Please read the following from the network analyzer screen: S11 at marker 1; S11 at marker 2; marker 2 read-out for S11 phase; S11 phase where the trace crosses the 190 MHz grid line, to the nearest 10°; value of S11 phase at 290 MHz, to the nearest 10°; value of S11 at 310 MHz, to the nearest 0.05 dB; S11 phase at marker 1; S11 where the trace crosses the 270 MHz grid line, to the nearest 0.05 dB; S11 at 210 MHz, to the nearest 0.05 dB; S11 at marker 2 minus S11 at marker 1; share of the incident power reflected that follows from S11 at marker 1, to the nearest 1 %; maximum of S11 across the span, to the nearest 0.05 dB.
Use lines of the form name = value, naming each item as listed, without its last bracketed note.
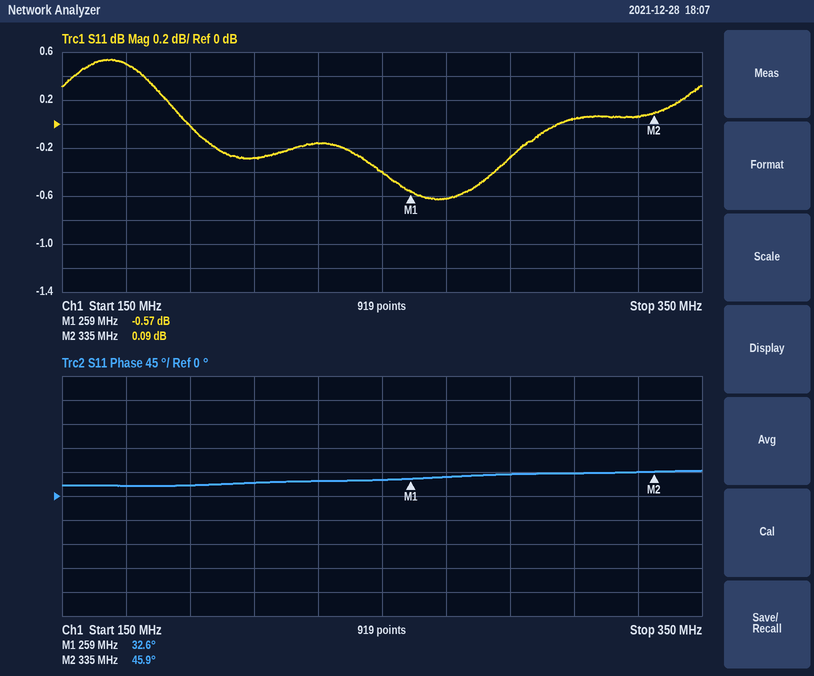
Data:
S11 at marker 1 = -0.57 dB
S11 at marker 2 = 0.09 dB
marker 2 read-out for S11 phase = 45.9°
S11 phase where the trace crosses the 190 MHz grid line, to the nearest 10° = 20°
value of S11 phase at 290 MHz, to the nearest 10° = 40°
value of S11 at 310 MHz, to the nearest 0.05 dB = 0.05 dB
S11 phase at marker 1 = 32.6°
S11 where the trace crosses the 270 MHz grid line, to the nearest 0.05 dB = -0.60 dB
S11 at 210 MHz, to the nearest 0.05 dB = -0.30 dB
S11 at marker 2 minus S11 at marker 1 = 0.66 dB
share of the incident power reflected that follows from S11 at marker 1, to the nearest 1 % = 88 %
maximum of S11 across the span, to the nearest 0.05 dB = 0.55 dB
